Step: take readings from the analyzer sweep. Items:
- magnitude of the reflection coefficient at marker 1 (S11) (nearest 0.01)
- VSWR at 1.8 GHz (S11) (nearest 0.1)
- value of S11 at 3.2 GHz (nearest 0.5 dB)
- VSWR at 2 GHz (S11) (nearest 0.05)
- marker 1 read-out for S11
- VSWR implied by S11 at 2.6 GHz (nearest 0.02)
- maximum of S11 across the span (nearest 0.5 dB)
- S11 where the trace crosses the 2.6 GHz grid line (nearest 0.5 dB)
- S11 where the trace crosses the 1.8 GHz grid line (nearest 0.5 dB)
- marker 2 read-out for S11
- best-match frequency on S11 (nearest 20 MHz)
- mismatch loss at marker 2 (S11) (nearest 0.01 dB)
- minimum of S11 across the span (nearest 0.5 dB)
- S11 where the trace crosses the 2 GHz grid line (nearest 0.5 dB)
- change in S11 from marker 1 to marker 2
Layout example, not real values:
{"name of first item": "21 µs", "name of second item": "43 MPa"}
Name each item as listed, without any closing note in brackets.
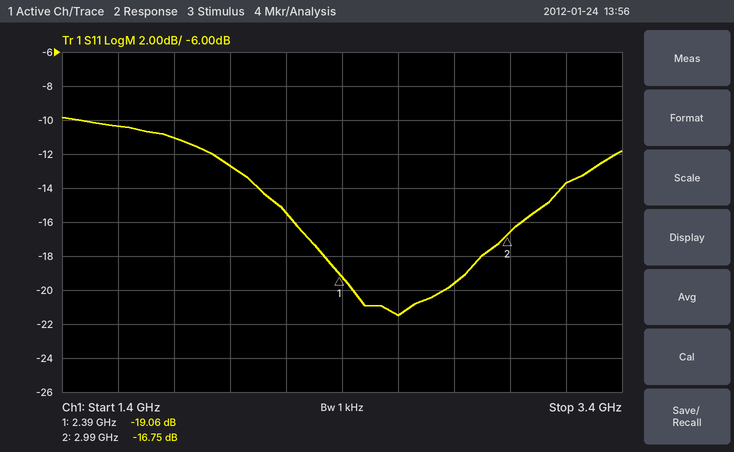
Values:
{"magnitude of the reflection coefficient at marker 1 (S11)": "0.11", "VSWR at 1.8 GHz (S11)": "1.8", "value of S11 at 3.2 GHz": "-13.5 dB", "VSWR at 2 GHz (S11)": "1.60", "marker 1 read-out for S11": "-19.06 dB", "VSWR implied by S11 at 2.6 GHz": "1.18", "maximum of S11 across the span": "-10.0 dB", "S11 where the trace crosses the 2.6 GHz grid line": "-21.5 dB", "S11 where the trace crosses the 1.8 GHz grid line": "-11.0 dB", "marker 2 read-out for S11": "-16.75 dB", "best-match frequency on S11": "2.60 GHz", "mismatch loss at marker 2 (S11)": "0.09 dB", "minimum of S11 across the span": "-21.5 dB", "S11 where the trace crosses the 2 GHz grid line": "-12.5 dB", "change in S11 from marker 1 to marker 2": "2.31 dB"}
